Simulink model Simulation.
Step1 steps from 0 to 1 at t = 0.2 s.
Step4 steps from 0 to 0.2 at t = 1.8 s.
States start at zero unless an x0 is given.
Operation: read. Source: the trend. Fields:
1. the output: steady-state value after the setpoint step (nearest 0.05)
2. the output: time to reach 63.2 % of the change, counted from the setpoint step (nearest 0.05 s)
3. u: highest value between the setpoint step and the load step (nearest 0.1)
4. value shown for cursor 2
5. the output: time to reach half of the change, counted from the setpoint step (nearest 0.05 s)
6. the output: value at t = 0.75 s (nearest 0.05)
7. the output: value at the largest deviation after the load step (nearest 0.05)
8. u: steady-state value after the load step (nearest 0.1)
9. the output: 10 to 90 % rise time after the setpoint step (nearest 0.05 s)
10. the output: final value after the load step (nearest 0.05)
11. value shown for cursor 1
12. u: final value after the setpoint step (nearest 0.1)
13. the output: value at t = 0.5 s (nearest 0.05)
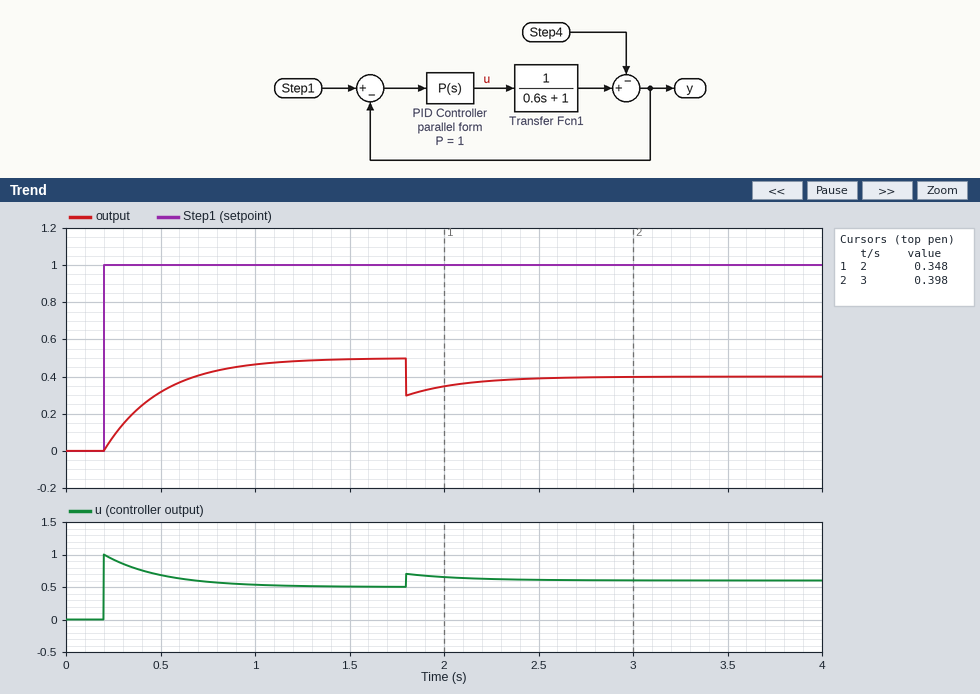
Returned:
0.50
0.30 s
1.0
0.398
0.20 s
0.40
0.30
0.6
0.65 s
0.40
0.348
0.5
0.30
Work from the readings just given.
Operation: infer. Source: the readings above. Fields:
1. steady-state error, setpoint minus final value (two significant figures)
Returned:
0.50
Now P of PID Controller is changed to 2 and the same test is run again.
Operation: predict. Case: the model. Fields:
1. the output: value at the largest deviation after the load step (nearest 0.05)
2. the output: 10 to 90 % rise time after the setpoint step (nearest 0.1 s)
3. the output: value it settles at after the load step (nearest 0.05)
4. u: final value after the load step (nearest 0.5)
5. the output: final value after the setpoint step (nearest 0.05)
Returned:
0.45
0.4 s
0.60
1.0
0.65
